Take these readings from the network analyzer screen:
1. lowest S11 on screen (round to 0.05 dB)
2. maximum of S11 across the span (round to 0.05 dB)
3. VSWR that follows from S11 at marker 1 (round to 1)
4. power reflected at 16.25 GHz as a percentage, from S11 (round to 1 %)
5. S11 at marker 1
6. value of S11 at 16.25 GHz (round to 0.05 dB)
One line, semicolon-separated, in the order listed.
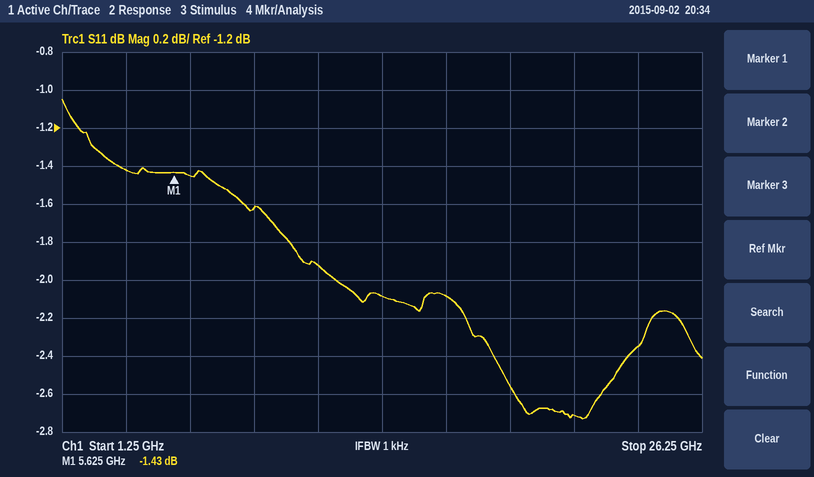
-2.75 dB; -1.05 dB; 12; 62 %; -1.43 dB; -2.10 dB
